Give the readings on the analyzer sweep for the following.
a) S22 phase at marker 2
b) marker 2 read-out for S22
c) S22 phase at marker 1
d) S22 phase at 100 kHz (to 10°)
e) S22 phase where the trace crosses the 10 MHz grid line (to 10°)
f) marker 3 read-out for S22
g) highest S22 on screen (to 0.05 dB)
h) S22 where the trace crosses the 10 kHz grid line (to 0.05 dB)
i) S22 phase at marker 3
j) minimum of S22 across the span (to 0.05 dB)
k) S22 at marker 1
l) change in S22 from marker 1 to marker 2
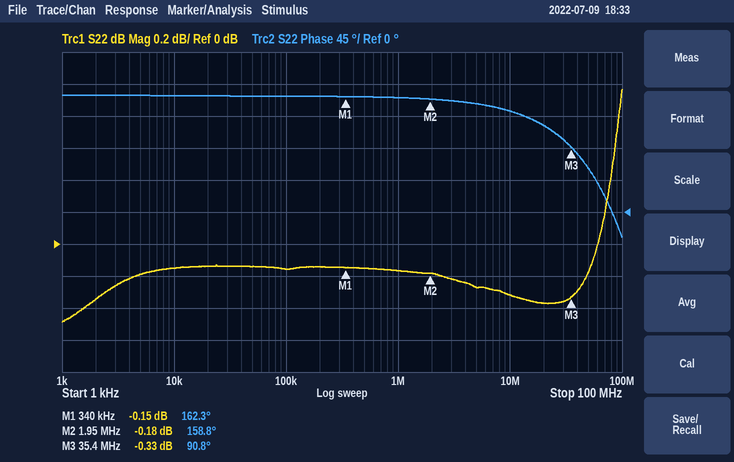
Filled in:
158.8°
-0.18 dB
162.3°
160°
140°
-0.33 dB
0.95 dB
-0.15 dB
90.8°
-0.50 dB
-0.15 dB
-0.03 dB
